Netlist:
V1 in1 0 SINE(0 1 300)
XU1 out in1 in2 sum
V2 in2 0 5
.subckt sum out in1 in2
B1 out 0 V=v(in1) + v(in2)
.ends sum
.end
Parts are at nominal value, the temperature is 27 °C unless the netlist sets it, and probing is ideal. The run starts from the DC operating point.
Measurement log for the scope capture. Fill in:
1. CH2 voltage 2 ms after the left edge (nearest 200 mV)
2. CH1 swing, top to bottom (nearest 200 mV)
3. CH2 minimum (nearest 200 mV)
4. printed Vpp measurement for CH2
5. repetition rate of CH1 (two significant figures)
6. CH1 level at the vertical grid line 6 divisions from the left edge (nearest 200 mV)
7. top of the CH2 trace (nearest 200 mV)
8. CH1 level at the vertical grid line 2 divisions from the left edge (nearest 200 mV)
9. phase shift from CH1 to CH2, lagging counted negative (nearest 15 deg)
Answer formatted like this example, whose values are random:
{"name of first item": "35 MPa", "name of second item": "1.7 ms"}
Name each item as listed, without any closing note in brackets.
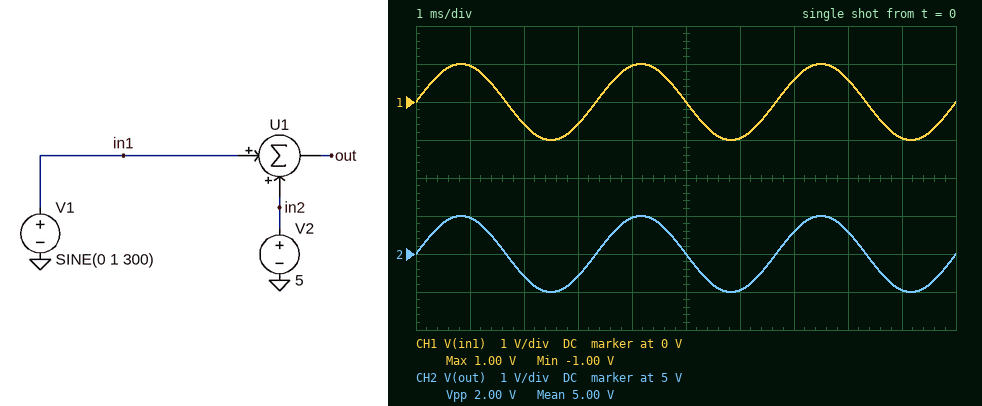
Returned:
{"CH2 voltage 2 ms after the left edge": "4.4 V", "CH1 swing, top to bottom": "2.0 V", "CH2 minimum": "4.0 V", "printed Vpp measurement for CH2": "2.00 V", "repetition rate of CH1": "300 Hz", "CH1 level at the vertical grid line 6 divisions from the left edge": "-1.0 V", "top of the CH2 trace": "6.0 V", "CH1 level at the vertical grid line 2 divisions from the left edge": "-600 mV", "phase shift from CH1 to CH2, lagging counted negative": "0 deg"}
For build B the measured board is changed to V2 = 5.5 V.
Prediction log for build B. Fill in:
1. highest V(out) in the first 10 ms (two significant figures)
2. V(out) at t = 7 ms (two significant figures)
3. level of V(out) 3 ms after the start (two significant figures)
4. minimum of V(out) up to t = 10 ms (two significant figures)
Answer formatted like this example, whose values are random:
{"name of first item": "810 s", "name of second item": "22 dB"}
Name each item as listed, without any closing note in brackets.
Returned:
{"highest V(out) in the first 10 ms": "6.5 V", "V(out) at t = 7 ms": "6.1 V", "level of V(out) 3 ms after the start": "4.9 V", "minimum of V(out) up to t = 10 ms": "4.5 V"}
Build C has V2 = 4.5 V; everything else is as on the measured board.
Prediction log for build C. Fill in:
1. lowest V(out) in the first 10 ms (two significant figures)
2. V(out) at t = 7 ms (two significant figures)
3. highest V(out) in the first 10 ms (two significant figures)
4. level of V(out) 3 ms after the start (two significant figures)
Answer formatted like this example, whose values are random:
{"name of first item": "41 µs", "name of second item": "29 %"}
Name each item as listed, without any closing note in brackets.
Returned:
{"lowest V(out) in the first 10 ms": "3.5 V", "V(out) at t = 7 ms": "5.1 V", "highest V(out) in the first 10 ms": "5.5 V", "level of V(out) 3 ms after the start": "3.9 V"}
